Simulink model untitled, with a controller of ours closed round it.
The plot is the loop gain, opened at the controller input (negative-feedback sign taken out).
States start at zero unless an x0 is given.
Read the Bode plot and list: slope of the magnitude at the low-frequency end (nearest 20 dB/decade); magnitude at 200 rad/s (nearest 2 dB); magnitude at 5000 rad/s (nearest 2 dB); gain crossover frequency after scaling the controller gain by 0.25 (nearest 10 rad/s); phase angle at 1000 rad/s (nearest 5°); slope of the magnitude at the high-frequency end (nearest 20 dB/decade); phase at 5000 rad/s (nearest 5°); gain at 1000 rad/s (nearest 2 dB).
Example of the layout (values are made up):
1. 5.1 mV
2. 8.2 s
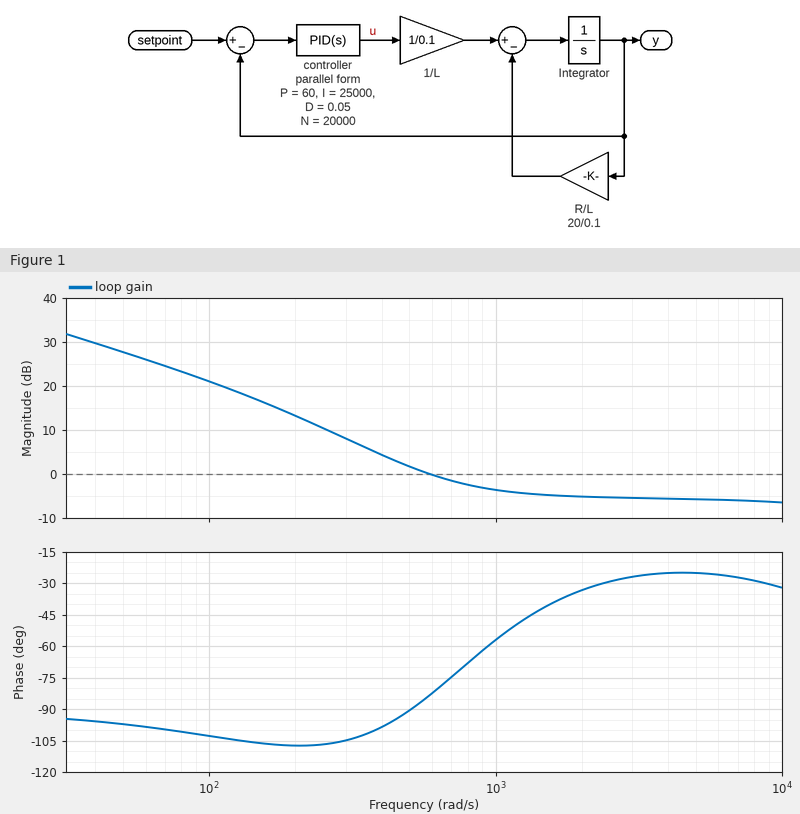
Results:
1. -20 dB/decade
2. 14 dB
3. -6 dB
4. 220 rad/s
5. -55°
6. 0 dB/decade
7. -25°
8. -4 dB
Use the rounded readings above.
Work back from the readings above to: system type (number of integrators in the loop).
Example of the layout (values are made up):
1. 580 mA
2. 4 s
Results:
1. 1
